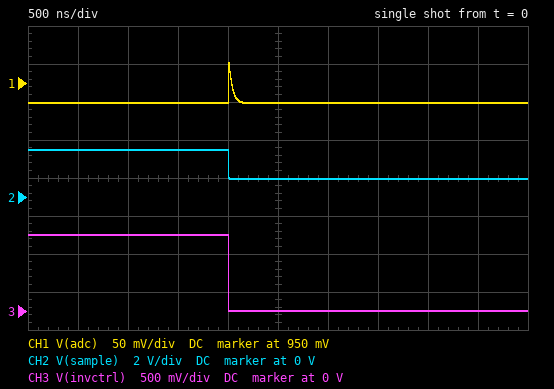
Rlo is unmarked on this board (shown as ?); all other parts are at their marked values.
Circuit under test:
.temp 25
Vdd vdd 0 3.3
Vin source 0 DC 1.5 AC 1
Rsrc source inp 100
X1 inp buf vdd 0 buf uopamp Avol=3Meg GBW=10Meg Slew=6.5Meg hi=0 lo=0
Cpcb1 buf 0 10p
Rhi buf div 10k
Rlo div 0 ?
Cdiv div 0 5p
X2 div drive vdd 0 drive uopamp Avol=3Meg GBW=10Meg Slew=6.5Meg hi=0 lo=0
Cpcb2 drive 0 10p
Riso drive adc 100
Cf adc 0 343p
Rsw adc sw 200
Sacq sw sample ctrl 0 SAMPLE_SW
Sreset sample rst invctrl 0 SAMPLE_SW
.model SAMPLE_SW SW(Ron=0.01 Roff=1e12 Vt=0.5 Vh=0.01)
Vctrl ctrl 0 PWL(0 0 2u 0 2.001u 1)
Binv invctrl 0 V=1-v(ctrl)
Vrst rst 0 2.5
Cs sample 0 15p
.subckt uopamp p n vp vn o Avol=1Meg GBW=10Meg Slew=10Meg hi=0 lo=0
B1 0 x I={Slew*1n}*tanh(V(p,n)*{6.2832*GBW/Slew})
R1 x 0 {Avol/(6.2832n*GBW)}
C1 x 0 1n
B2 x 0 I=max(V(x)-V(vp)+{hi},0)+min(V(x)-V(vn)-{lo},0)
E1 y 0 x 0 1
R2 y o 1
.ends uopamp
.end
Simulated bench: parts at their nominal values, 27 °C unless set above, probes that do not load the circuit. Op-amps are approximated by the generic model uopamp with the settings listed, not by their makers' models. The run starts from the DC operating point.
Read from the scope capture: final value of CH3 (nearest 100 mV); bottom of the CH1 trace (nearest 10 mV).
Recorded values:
0 V
920 mV
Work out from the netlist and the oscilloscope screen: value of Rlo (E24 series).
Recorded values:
16 kΩ
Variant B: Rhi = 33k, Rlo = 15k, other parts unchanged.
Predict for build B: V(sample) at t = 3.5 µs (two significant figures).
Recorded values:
470 mV
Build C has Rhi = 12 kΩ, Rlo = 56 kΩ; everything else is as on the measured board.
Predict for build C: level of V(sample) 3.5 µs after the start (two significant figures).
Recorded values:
1.2 V
